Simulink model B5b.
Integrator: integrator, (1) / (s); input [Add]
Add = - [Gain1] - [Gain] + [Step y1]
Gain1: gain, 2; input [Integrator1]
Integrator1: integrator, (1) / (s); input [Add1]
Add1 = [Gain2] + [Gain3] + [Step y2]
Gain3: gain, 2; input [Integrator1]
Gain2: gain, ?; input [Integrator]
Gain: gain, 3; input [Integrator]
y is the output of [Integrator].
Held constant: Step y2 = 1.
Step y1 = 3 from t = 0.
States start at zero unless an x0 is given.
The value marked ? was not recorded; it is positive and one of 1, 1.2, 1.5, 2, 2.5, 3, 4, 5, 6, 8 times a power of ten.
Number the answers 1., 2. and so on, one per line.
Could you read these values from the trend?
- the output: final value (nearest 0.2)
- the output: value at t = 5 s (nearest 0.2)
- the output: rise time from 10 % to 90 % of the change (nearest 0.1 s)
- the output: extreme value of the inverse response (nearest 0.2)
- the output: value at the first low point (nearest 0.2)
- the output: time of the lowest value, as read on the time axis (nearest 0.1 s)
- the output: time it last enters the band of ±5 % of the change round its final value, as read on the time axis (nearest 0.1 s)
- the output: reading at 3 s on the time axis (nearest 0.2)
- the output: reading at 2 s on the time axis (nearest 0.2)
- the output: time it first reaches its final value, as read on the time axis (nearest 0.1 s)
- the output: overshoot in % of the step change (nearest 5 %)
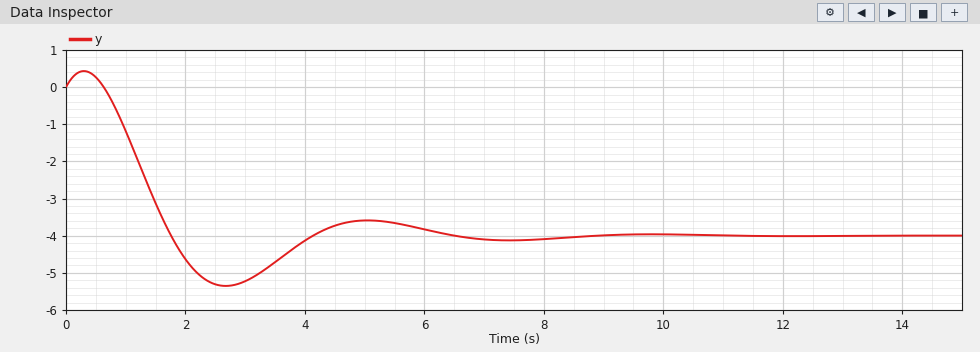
1. -4.0
2. -3.6
3. 0.9 s
4. 0.4
5. -5.4
6. 2.7 s
7. 5.9 s
8. -5.2
9. -4.6
10. 1.8 s
11. 35 %
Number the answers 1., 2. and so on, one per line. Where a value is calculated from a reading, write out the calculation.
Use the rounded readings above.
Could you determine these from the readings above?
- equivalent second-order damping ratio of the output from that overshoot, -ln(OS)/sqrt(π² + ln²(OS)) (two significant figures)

1. ln(0.35) = -1.050; 1.050 / sqrt(9.870 + 1.102) = 0.32
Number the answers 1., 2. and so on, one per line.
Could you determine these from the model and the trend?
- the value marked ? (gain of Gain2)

1. 4
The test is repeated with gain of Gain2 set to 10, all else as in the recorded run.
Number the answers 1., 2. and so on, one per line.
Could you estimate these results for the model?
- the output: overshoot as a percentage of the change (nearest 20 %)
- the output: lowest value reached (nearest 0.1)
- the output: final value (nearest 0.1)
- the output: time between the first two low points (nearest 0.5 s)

1. 100 %
2. -1.2
3. -0.6
4. 1.5 s
